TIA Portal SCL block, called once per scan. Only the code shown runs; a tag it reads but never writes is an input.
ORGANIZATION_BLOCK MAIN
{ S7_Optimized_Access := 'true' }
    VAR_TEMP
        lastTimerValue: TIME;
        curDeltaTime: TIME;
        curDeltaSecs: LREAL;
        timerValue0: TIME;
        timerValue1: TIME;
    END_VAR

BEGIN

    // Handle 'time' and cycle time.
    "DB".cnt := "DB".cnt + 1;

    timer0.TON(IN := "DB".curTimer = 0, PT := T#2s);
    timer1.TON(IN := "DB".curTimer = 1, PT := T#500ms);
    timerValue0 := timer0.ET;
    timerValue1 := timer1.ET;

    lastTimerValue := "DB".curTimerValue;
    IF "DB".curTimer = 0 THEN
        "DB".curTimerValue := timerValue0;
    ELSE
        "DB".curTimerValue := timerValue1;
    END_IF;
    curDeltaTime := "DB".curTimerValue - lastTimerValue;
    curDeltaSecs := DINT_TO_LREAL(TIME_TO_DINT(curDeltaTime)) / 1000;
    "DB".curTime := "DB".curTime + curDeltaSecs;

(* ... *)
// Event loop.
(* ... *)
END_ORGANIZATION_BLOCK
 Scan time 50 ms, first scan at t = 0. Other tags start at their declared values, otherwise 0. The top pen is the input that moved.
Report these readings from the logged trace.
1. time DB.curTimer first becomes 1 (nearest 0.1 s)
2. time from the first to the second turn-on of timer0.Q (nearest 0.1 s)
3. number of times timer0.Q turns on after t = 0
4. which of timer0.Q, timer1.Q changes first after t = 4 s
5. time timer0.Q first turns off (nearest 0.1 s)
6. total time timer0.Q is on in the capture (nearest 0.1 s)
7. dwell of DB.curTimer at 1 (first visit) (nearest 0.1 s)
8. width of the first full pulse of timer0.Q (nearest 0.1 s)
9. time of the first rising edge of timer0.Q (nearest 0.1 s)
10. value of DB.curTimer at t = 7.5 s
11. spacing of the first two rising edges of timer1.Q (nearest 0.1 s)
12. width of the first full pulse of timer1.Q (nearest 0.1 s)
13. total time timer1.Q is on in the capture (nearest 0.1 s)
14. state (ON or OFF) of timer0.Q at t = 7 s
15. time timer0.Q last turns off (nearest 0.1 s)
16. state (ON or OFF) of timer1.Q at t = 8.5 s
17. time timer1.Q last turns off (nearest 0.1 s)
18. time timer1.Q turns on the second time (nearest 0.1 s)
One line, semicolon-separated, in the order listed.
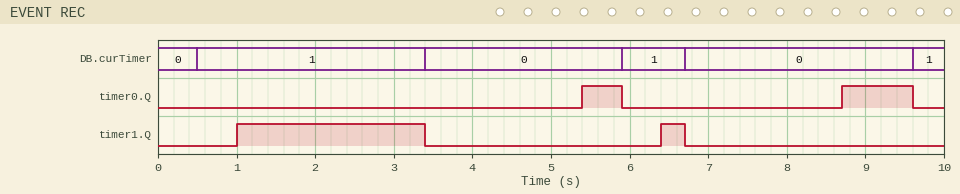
0.5 s; 3.3 s; 2; timer0.Q; 5.9 s; 1.4 s; 2.9 s; 0.5 s; 5.4 s; 0; 5.4 s; 2.4 s; 2.7 s; OFF; 9.6 s; OFF; 6.7 s; 6.4 s
